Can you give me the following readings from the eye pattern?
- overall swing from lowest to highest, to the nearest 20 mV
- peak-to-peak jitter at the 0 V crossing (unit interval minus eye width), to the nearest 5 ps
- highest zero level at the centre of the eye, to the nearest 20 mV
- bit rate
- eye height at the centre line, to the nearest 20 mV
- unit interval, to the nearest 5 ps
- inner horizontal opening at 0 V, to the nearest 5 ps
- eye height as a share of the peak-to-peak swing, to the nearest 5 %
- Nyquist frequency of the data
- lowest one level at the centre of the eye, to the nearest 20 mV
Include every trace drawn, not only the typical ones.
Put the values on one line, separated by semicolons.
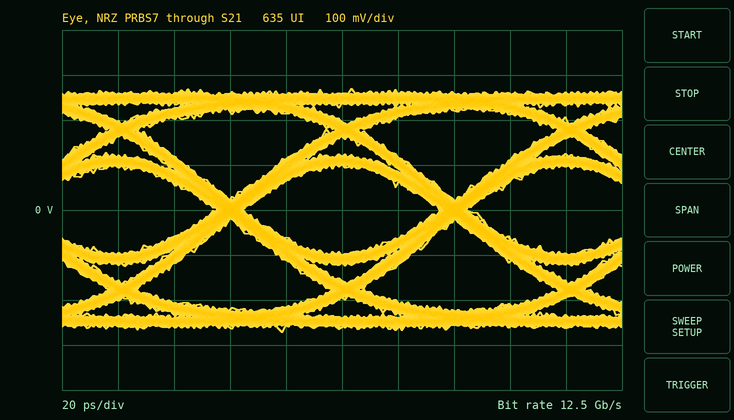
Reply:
540 mV; 10 ps; -100 mV; 12.5 Gb/s; 200 mV; 80 ps; 70 ps; 35 %; 6.25 GHz; 100 mV
